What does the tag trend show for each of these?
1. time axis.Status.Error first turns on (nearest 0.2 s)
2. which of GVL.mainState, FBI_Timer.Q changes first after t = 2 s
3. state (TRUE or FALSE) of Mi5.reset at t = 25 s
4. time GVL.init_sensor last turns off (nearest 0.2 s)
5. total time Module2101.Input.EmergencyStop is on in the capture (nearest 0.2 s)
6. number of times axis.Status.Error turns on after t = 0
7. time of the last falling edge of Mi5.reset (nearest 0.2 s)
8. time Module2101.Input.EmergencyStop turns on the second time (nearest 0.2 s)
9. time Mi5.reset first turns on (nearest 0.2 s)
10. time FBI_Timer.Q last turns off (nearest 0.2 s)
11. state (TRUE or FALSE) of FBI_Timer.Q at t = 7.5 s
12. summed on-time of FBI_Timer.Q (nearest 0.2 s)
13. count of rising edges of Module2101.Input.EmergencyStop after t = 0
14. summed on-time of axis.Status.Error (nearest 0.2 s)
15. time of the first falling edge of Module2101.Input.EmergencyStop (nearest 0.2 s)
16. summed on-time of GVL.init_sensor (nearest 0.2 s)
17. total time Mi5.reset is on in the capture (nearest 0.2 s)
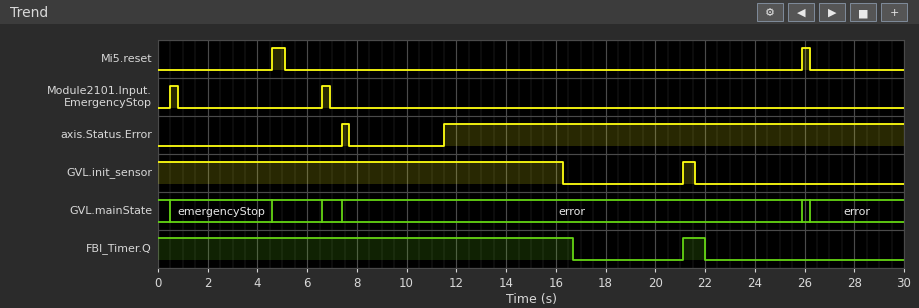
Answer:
7.4 s
GVL.mainState
FALSE
21.6 s
0.6 s
2
26.2 s
6.6 s
4.6 s
22.0 s
TRUE
17.6 s
2
18.8 s
0.8 s
16.8 s
0.8 s
